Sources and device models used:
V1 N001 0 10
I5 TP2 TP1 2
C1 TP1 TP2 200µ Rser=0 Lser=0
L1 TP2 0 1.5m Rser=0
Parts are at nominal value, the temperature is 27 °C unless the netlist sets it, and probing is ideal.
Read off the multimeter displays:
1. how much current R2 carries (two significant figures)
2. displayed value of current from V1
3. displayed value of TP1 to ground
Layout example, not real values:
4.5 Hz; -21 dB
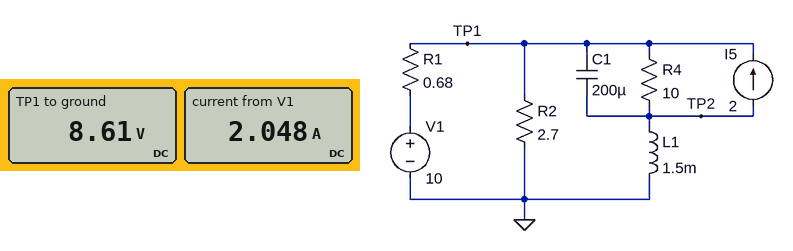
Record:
3.2 A; 2.048 A; 8.61 V
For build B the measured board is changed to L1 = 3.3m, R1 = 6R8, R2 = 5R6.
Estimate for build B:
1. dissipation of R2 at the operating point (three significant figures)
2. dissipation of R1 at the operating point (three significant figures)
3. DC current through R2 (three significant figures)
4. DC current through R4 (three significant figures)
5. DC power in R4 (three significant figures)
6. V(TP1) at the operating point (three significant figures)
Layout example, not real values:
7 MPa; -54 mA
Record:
11.9 W; 501 mW; 1.46 A; 815 mA; 6.65 W; 8.15 V
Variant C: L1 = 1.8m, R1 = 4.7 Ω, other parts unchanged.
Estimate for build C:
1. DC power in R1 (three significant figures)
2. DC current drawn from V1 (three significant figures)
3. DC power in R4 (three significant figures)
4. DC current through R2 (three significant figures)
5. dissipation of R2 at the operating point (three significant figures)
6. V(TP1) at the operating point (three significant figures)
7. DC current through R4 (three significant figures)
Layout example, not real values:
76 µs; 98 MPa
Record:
3.33 W; 842 mA; 3.65 W; 2.24 A; 13.5 W; 6.04 V; 604 mA
